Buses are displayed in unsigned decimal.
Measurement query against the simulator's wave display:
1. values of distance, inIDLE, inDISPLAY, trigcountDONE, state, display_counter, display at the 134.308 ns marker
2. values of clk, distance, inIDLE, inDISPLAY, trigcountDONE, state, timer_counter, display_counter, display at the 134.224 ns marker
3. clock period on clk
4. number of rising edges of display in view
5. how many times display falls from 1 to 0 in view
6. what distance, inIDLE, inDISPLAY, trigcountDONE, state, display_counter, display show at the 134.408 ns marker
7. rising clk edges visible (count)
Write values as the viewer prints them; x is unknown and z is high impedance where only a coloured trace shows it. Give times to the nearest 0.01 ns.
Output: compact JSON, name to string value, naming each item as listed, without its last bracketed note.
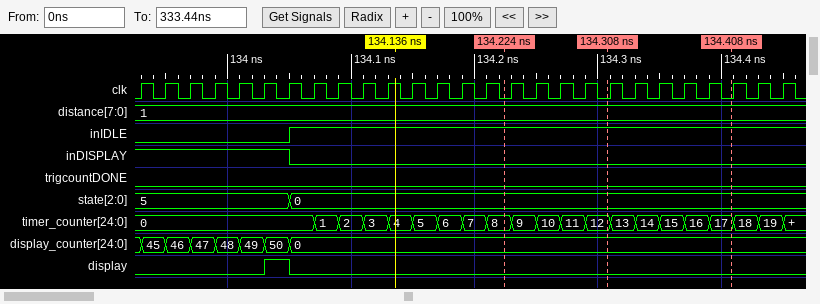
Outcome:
{"values of distance, inIDLE, inDISPLAY, trigcountDONE, state, display_counter, display at the 134.308 ns marker": "distance=1, inIDLE=1, inDISPLAY=0, trigcountDONE=0, state=0, display_counter=0, display=0", "values of clk, distance, inIDLE, inDISPLAY, trigcountDONE, state, timer_counter, display_counter, display at the 134.224 ns marker": "clk=0, distance=1, inIDLE=1, inDISPLAY=0, trigcountDONE=0, state=0, timer_counter=8, display_counter=0, display=0", "clock period on clk": "0.02 ns", "number of rising edges of display in view": "1", "how many times display falls from 1 to 0 in view": "1", "what distance, inIDLE, inDISPLAY, trigcountDONE, state, display_counter, display show at the 134.408 ns marker": "distance=1, inIDLE=1, inDISPLAY=0, trigcountDONE=0, state=0, display_counter=0, display=0", "rising clk edges visible": "27"}
